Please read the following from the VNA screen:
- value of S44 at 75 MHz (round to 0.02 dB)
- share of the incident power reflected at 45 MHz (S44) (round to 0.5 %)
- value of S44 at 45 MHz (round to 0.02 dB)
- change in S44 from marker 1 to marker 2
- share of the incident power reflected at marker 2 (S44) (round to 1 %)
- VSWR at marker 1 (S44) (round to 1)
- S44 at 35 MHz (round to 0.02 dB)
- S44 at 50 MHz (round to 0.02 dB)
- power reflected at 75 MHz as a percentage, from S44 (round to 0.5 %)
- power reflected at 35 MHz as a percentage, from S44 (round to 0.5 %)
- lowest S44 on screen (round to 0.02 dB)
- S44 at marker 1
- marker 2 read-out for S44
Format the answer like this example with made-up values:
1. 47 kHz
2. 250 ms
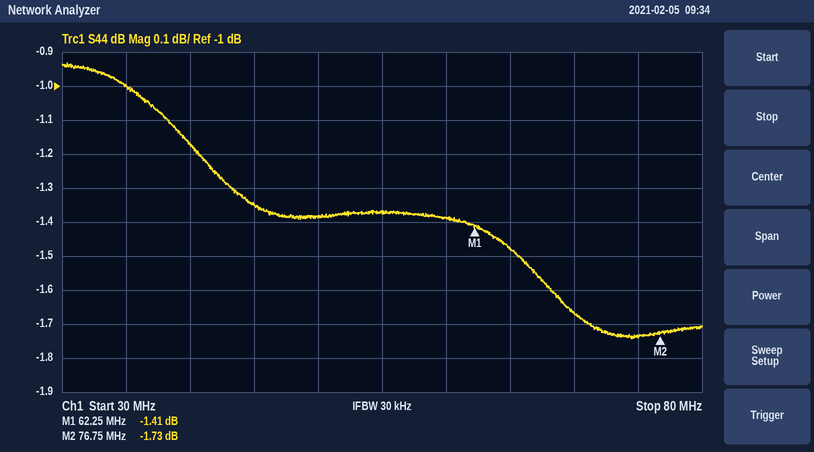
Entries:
1. -1.74 dB
2. 73.5 %
3. -1.34 dB
4. -0.32 dB
5. 67 %
6. 12
7. -1.00 dB
8. -1.38 dB
9. 67.0 %
10. 79.5 %
11. -1.74 dB
12. -1.41 dB
13. -1.73 dB
